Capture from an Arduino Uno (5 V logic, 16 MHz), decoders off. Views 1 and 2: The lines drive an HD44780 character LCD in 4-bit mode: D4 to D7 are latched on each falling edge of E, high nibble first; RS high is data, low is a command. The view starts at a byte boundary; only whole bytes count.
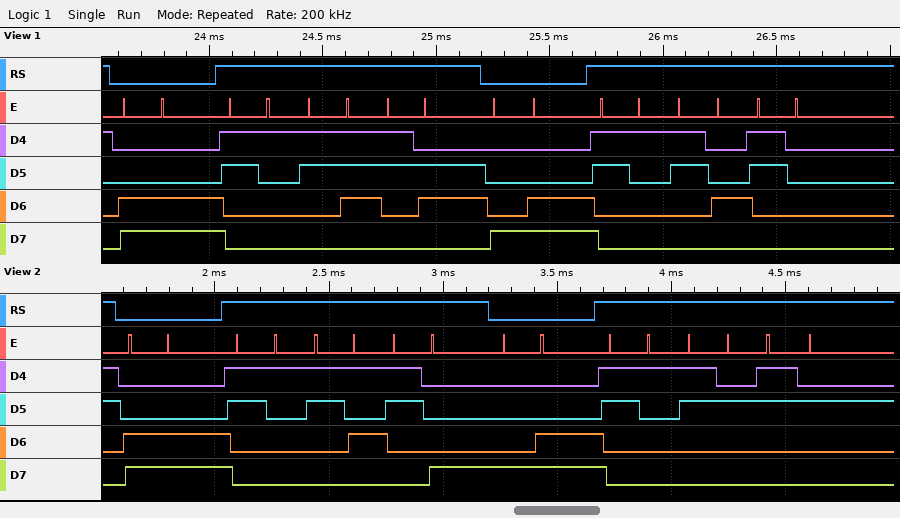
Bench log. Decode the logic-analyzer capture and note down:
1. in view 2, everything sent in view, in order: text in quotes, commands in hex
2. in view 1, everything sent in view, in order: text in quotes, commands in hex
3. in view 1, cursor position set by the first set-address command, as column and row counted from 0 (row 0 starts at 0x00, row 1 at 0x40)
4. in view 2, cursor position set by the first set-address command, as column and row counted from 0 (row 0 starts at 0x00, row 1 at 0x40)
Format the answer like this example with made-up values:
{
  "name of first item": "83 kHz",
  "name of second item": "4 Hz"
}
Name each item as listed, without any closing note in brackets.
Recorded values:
{
  "in view 2, everything sent in view, in order: text in quotes, commands in hex": "0xCC \"158\" 0x8C \"122\"",
  "in view 1, everything sent in view, in order: text in quotes, commands in hex": "0xCC \"176\" 0x8C \"140\"",
  "in view 1, cursor position set by the first set-address command, as column and row counted from 0": "column 12, row 1",
  "in view 2, cursor position set by the first set-address command, as column and row counted from 0": "column 12, row 1"
}
